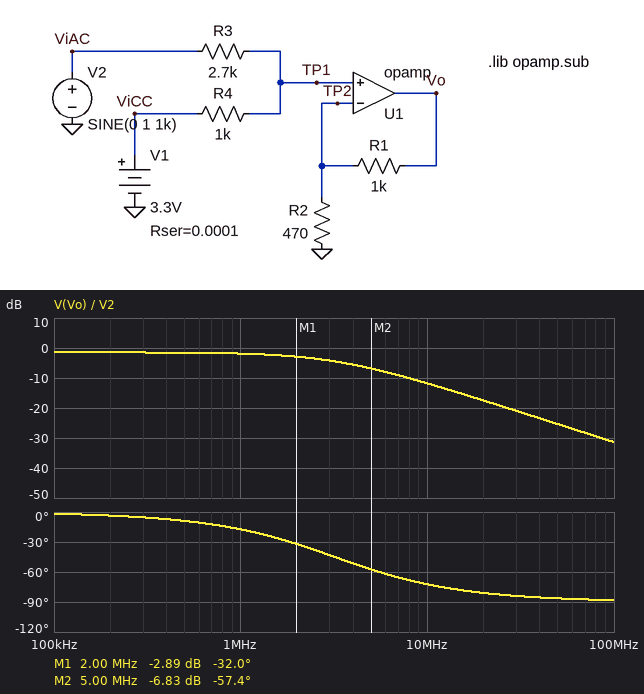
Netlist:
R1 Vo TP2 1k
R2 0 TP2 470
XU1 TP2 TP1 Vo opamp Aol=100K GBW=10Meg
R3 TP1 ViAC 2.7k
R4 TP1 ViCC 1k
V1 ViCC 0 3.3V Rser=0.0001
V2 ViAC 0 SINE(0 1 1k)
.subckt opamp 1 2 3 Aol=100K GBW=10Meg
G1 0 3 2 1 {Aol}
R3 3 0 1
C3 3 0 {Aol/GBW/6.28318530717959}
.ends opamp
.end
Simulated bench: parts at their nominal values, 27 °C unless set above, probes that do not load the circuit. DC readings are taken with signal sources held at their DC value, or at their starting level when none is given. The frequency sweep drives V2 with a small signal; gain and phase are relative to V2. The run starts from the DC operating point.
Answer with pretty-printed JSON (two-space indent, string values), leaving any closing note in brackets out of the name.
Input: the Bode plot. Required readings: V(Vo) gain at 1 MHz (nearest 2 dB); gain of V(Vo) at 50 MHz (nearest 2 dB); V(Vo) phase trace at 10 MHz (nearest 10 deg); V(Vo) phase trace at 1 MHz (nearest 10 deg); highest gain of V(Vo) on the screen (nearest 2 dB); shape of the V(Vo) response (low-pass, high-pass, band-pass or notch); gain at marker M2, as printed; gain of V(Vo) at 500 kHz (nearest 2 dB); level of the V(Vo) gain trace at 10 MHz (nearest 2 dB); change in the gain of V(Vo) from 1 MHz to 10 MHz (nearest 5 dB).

{
  "V(Vo) gain at 1 MHz": "-2 dB",
  "gain of V(Vo) at 50 MHz": "-26 dB",
  "V(Vo) phase trace at 10 MHz": "-70 deg",
  "V(Vo) phase trace at 1 MHz": "-20 deg",
  "highest gain of V(Vo) on the screen": "-2 dB",
  "shape of the V(Vo) response": "low-pass",
  "gain at marker M2, as printed": "-6.83 dB",
  "gain of V(Vo) at 500 kHz": "-2 dB",
  "level of the V(Vo) gain trace at 10 MHz": "-12 dB",
  "change in the gain of V(Vo) from 1 MHz to 10 MHz": "-10 dB"
}
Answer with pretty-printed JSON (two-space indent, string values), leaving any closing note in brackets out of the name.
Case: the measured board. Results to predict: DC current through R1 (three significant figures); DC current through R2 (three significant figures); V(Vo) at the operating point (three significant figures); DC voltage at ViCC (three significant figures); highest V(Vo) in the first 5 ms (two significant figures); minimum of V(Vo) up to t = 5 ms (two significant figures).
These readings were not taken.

{
  "DC current through R1": "5.12 mA",
  "DC current through R2": "5.12 mA",
  "V(Vo) at the operating point": "7.53 V",
  "DC voltage at ViCC": "3.30 V",
  "highest V(Vo) in the first 5 ms": "8.4 V",
  "minimum of V(Vo) up to t = 5 ms": "6.7 V"
}
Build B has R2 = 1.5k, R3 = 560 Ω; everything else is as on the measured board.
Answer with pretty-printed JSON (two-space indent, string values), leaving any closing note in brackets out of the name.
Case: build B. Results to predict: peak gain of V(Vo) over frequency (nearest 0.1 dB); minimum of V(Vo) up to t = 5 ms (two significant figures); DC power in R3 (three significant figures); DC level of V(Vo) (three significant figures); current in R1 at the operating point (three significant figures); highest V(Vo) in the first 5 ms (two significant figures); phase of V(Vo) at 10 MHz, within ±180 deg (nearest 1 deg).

{
  "peak gain of V(Vo) over frequency": "0.6 dB",
  "minimum of V(Vo) up to t = 5 ms": "910 mV",
  "DC power in R3": "2.51 mW",
  "DC level of V(Vo)": "1.97 V",
  "current in R1 at the operating point": "790 µA",
  "highest V(Vo) in the first 5 ms": "3.0 V",
  "phase of V(Vo) at 10 MHz, within ±180 deg": "-59 deg"
}
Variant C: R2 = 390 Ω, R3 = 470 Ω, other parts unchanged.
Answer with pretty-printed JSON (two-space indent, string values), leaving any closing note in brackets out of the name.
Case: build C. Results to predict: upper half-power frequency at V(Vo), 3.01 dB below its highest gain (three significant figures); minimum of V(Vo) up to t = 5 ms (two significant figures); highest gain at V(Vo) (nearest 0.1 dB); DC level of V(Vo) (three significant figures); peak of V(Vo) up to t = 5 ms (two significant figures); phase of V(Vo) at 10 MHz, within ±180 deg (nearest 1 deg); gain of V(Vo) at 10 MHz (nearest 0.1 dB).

{
  "upper half-power frequency at V(Vo), 3.01 dB below its highest gain": "2.81 MHz",
  "minimum of V(Vo) up to t = 5 ms": "1.3 V",
  "highest gain at V(Vo)": "7.7 dB",
  "DC level of V(Vo)": "3.76 V",
  "peak of V(Vo) up to t = 5 ms": "6.2 V",
  "phase of V(Vo) at 10 MHz, within ±180 deg": "-74 deg",
  "gain of V(Vo) at 10 MHz": "-3.7 dB"
}
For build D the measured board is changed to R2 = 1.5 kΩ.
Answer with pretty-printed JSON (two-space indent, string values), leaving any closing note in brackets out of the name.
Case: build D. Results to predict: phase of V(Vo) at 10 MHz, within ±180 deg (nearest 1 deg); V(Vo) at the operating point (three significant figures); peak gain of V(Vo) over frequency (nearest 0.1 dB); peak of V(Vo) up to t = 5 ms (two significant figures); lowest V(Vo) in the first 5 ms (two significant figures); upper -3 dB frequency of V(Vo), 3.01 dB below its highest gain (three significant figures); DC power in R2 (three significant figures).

{
  "phase of V(Vo) at 10 MHz, within ±180 deg": "-59 deg",
  "V(Vo) at the operating point": "4.01 V",
  "peak gain of V(Vo) over frequency": "-6.9 dB",
  "peak of V(Vo) up to t = 5 ms": "4.5 V",
  "lowest V(Vo) in the first 5 ms": "3.6 V",
  "upper -3 dB frequency of V(Vo), 3.01 dB below its highest gain": "6.00 MHz",
  "DC power in R2": "3.87 mW"
}
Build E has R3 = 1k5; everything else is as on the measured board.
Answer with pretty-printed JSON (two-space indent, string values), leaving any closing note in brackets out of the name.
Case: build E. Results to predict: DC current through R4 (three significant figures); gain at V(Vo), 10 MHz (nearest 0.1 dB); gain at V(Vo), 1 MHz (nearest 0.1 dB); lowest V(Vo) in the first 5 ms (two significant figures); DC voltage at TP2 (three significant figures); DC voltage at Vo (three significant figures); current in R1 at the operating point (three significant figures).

{
  "DC current through R4": "1.32 mA",
  "gain at V(Vo), 10 MHz": "-8.4 dB",
  "gain at V(Vo), 1 MHz": "1.5 dB",
  "lowest V(Vo) in the first 5 ms": "4.9 V",
  "DC voltage at TP2": "1.98 V",
  "DC voltage at Vo": "6.19 V",
  "current in R1 at the operating point": "4.21 mA"
}
